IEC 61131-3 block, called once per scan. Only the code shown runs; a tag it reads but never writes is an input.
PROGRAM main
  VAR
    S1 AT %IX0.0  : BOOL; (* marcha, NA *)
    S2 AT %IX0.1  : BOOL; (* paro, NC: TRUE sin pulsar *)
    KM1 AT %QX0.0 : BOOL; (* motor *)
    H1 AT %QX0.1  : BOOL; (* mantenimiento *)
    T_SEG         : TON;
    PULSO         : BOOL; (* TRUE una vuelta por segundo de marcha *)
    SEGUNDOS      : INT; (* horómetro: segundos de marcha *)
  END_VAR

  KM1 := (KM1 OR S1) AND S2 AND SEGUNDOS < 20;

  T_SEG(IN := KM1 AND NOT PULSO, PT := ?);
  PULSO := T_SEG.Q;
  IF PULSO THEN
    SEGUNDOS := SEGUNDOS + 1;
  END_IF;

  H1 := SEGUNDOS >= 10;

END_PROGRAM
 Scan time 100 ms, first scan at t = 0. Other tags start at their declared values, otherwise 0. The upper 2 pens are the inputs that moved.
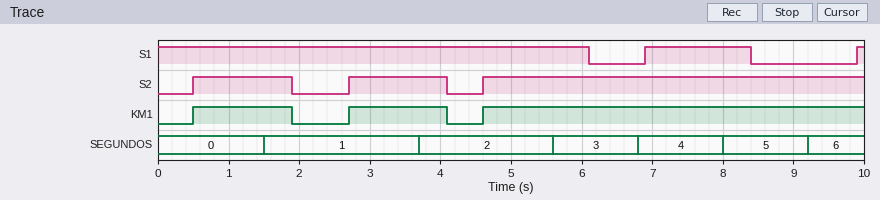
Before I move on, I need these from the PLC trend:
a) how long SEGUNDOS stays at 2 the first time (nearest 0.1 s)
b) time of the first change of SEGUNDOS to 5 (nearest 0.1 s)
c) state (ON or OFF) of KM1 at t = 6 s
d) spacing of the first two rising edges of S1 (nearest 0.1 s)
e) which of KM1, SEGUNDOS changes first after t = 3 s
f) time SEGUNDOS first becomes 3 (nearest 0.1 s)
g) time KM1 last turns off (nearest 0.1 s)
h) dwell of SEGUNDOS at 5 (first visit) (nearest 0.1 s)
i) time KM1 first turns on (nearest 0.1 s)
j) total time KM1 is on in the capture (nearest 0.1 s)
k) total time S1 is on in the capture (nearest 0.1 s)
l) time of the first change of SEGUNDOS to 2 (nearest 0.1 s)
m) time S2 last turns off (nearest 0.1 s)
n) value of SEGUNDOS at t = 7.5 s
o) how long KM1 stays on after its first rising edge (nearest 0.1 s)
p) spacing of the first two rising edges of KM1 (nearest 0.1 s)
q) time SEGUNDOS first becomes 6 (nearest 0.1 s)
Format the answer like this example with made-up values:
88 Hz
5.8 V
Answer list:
1.9 s
8.0 s
ON
3.0 s
SEGUNDOS
5.6 s
4.1 s
1.2 s
0.5 s
8.2 s
7.7 s
3.7 s
4.1 s
4
1.4 s
2.2 s
9.2 s
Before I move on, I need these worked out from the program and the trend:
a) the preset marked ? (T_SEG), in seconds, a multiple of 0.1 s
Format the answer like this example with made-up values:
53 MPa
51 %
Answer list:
1.0 s
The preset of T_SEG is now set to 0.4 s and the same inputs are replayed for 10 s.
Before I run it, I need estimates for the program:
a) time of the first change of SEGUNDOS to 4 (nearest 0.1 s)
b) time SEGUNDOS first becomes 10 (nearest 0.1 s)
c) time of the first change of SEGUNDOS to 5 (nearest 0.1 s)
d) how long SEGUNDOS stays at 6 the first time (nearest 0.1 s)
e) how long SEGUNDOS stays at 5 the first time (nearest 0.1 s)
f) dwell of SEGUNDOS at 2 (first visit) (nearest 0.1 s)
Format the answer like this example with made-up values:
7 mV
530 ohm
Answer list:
3.7 s
8.0 s
5.0 s
0.6 s
0.6 s
1.6 s
